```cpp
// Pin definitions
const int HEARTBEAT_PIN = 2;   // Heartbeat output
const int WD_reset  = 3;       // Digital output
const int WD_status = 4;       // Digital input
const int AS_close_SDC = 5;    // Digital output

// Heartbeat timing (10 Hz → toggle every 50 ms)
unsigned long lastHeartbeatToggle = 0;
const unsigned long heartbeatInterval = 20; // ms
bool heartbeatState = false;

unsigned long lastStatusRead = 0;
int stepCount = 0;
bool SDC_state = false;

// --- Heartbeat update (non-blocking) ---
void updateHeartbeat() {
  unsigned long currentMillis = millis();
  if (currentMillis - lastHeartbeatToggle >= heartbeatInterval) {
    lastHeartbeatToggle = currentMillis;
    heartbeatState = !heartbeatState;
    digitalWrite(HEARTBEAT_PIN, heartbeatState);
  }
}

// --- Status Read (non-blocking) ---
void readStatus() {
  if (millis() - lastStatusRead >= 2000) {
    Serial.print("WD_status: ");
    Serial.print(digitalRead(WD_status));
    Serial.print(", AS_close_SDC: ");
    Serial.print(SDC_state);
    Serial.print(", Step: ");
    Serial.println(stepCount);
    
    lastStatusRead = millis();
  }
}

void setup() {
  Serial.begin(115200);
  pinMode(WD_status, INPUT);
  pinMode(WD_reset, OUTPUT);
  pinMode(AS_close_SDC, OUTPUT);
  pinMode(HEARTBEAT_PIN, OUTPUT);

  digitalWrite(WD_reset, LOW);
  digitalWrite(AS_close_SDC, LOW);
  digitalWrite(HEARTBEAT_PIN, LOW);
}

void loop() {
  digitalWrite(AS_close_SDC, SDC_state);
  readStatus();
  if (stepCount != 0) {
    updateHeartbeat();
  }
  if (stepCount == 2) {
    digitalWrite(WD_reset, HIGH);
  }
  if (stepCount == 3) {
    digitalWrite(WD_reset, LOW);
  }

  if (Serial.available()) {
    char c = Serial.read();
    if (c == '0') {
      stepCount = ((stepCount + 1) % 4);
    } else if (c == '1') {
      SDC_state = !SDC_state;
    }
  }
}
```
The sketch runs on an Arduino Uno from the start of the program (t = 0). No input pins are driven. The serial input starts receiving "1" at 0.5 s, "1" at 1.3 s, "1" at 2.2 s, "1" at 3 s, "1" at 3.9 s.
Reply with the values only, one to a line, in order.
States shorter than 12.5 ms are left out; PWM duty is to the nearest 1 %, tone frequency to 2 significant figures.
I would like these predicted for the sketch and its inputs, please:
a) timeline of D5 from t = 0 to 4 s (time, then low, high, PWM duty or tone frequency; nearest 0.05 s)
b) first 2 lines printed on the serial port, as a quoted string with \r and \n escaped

0 s low; 0.5 s high; 1.3 s low; 2.2 s high; 3 s low; 3.9 s high
"WD_status: 0, AS_close_SDC: 0, Step: 0\r\nWD_status: 0, AS_close_SDC: 1, Step: 0\r\n"
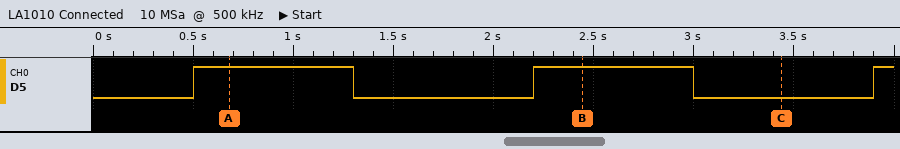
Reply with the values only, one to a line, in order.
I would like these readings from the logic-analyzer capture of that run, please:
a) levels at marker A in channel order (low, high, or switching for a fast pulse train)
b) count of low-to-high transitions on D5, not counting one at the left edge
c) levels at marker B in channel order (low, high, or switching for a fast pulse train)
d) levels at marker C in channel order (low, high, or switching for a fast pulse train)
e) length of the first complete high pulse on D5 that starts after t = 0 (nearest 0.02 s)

D5 high
3
D5 high
D5 low
0.80 s
